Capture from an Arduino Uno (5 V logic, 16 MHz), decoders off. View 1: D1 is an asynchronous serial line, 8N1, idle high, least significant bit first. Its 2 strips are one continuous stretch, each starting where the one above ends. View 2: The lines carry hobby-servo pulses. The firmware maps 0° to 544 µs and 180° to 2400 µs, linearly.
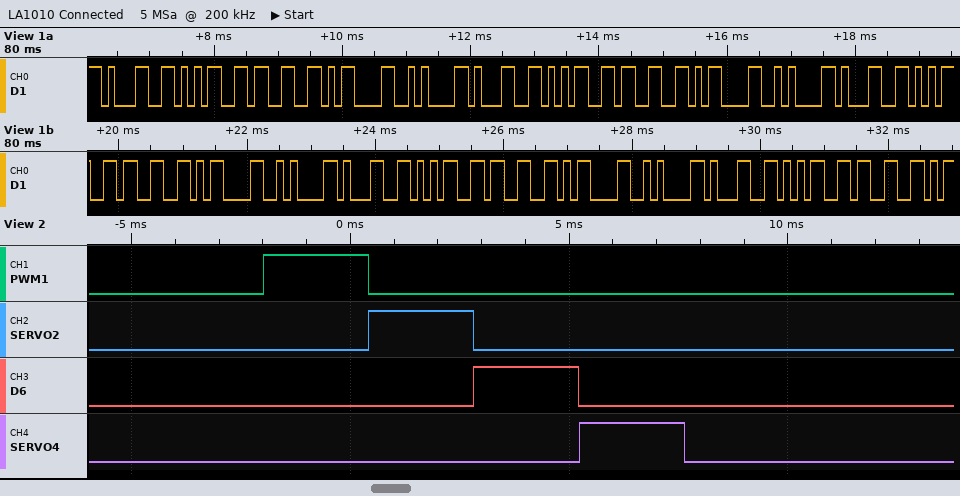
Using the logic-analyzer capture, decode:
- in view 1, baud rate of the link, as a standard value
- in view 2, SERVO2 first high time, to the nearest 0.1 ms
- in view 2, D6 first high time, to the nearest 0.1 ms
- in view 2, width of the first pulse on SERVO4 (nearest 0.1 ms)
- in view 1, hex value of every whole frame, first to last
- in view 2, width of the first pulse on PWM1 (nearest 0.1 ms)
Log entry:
9600 baud
2.4 ms
2.4 ms
2.4 ms
0x31 0x35 0x33 0x0D 0x0A 0x31 0x35 0x33 0x0D 0x0A 0x31 0x35 0x33 0x0D 0x0A 0x31 0x35 0x33 0x0D 0x0A 0x31 0x35 0x33
2.4 ms
